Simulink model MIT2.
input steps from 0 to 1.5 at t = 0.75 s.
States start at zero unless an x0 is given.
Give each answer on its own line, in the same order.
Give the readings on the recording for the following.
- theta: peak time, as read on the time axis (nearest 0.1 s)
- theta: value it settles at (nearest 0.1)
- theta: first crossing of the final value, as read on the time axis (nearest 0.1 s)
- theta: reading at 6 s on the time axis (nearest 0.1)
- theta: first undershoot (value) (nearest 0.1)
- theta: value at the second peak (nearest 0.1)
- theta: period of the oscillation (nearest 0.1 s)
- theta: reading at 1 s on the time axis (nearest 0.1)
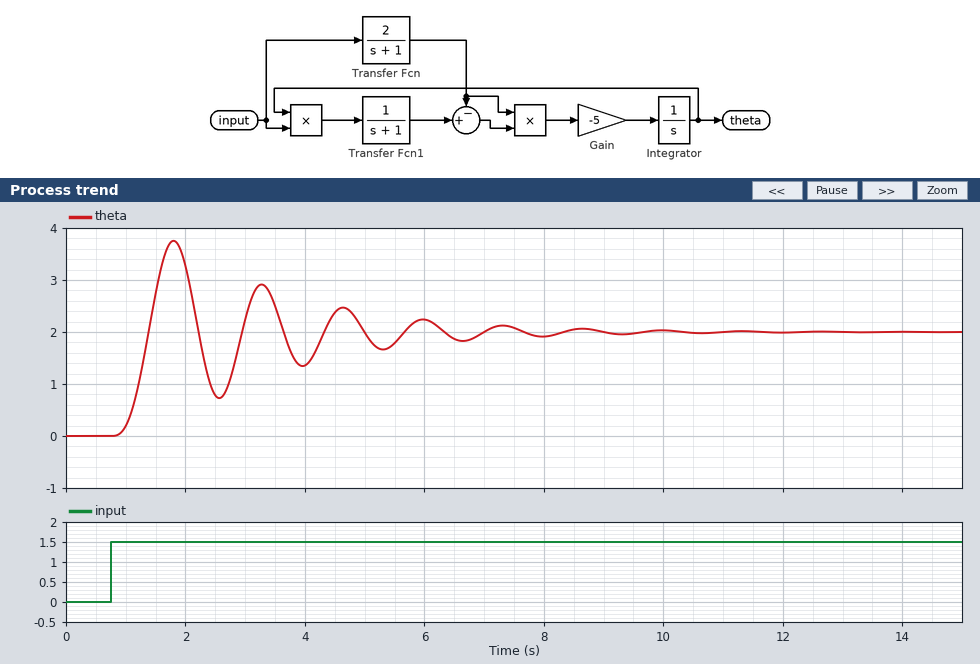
1.8 s
2.0
1.4 s
2.2
0.7
2.9
1.5 s
0.2
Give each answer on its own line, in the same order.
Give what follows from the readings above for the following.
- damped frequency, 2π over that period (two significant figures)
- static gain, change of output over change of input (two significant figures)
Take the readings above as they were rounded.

4.2 rad/s
1.3
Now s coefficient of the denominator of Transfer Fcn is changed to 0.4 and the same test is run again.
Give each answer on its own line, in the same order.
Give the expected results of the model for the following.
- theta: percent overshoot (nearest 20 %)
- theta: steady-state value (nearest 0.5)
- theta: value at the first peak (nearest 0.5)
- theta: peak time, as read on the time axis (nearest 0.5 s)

200 %
2.0
6.0
1.5 s
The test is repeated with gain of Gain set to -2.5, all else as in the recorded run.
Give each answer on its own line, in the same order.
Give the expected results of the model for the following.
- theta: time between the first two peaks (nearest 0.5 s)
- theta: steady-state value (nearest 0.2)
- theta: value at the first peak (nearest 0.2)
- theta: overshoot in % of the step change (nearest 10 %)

2.0 s
2.0
3.4
70 %
